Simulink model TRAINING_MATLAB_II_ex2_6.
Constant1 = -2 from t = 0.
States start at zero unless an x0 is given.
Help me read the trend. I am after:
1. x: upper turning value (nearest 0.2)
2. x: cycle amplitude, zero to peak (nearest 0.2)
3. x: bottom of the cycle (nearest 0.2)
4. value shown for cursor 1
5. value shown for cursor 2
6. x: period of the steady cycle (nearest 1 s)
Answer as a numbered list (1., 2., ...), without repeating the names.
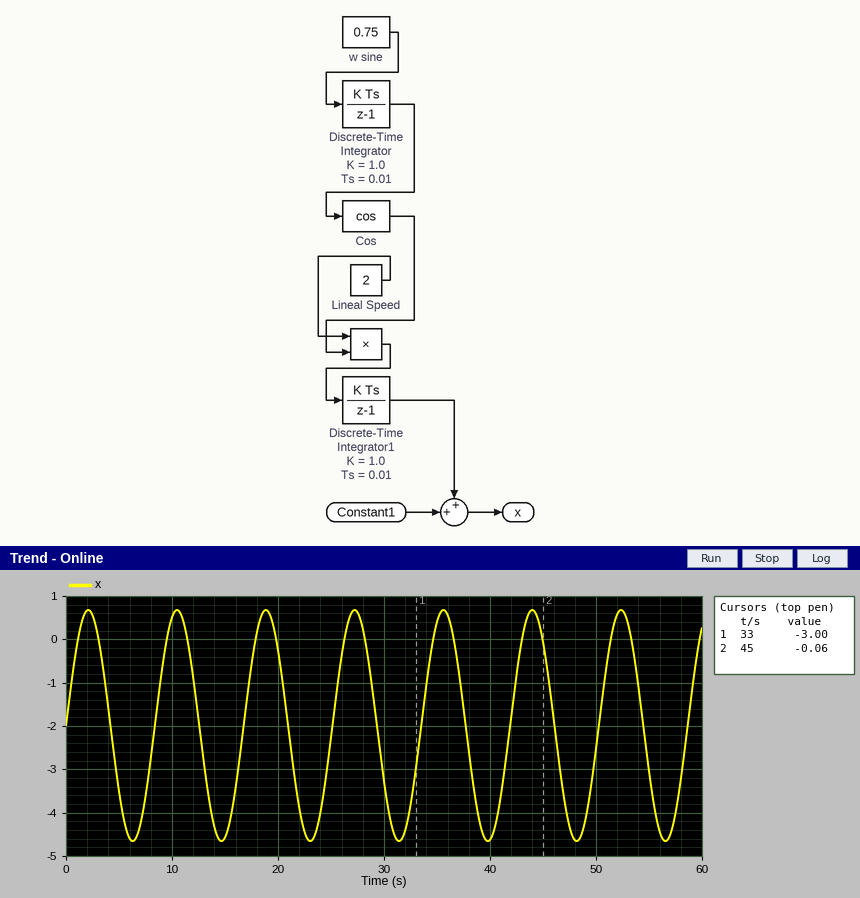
1. 0.6
2. 2.6
3. -4.6
4. -3.00
5. -0.06
6. 8 s
